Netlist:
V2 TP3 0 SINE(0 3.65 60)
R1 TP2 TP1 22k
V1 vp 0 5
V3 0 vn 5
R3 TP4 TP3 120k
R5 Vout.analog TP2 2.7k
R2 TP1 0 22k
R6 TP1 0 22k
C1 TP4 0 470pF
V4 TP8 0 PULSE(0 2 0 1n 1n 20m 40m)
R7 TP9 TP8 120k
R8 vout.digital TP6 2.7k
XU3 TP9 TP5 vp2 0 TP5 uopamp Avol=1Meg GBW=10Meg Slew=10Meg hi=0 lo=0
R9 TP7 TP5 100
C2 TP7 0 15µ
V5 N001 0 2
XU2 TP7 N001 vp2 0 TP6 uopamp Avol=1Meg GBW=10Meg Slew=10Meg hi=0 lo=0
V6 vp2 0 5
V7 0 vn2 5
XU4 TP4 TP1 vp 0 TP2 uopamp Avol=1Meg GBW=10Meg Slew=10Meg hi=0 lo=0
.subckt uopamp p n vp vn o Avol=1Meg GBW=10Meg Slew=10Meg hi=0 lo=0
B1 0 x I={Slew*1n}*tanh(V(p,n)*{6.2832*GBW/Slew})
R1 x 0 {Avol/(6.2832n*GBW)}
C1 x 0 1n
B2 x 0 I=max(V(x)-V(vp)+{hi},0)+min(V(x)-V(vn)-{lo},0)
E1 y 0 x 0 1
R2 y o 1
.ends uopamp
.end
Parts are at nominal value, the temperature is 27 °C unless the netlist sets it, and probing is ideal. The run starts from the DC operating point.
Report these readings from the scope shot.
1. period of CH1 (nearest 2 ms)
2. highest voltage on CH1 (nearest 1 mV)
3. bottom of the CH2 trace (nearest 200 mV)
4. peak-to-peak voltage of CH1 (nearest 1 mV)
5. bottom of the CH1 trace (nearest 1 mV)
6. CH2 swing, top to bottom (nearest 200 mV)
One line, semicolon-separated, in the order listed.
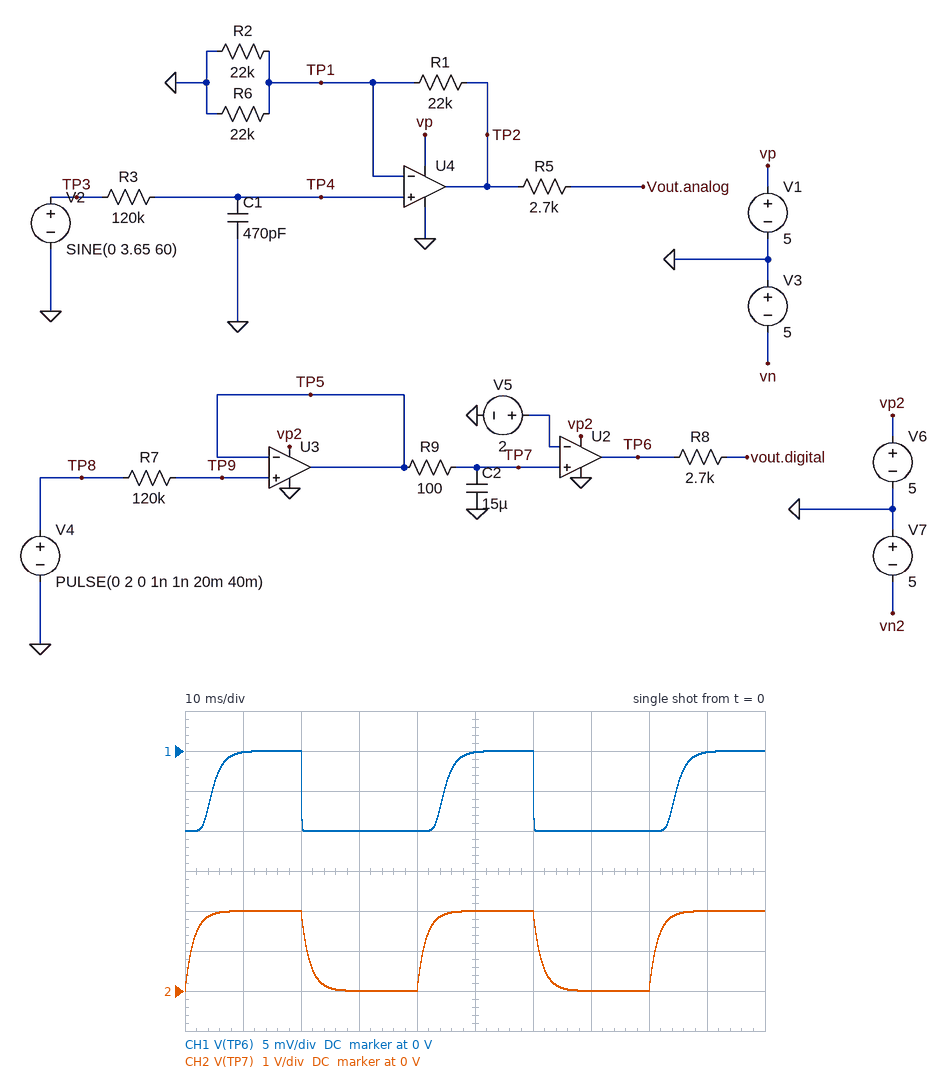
40 ms; 0 V; 0 V; 10 mV; -10 mV; 2.0 V
